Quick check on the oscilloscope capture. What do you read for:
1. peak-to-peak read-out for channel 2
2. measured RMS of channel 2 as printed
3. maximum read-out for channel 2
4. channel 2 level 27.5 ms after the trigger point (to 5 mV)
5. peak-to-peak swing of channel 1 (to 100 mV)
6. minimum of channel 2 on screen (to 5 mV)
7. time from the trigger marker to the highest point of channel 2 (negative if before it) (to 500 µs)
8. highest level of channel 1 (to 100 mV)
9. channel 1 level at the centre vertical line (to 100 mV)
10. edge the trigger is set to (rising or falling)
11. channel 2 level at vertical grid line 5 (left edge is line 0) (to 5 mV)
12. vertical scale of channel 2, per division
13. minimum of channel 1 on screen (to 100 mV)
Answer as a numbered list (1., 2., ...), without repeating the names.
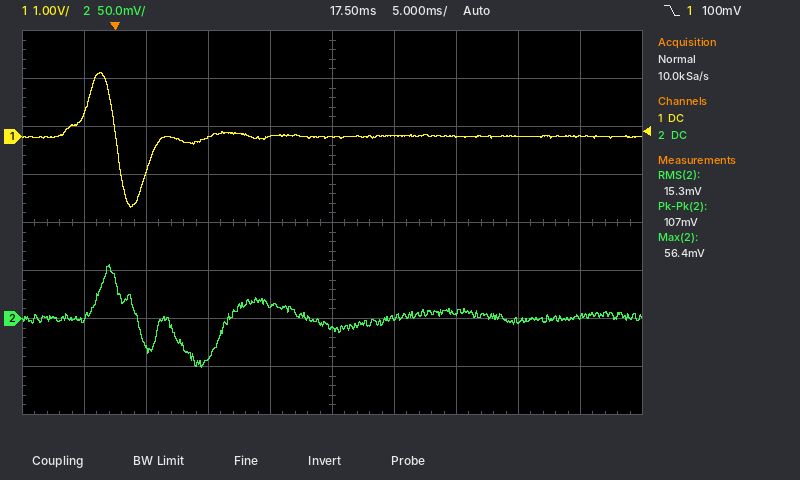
1. 107 mV
2. 15.3 mV
3. 56.4 mV
4. 5 mV
5. 2.8 V
6. -50 mV
7. -500 µs
8. 1.3 V
9. 0.0 V
10. falling
11. -10 mV
12. 50 mV
13. -1.5 V
